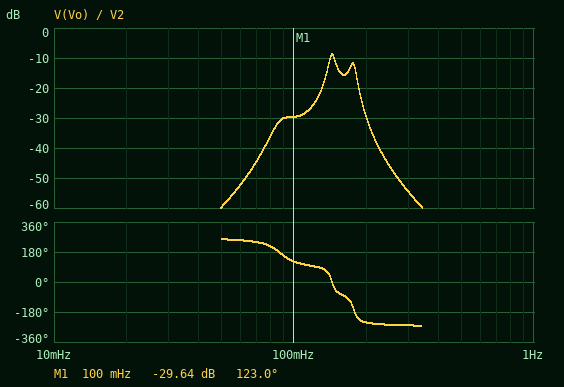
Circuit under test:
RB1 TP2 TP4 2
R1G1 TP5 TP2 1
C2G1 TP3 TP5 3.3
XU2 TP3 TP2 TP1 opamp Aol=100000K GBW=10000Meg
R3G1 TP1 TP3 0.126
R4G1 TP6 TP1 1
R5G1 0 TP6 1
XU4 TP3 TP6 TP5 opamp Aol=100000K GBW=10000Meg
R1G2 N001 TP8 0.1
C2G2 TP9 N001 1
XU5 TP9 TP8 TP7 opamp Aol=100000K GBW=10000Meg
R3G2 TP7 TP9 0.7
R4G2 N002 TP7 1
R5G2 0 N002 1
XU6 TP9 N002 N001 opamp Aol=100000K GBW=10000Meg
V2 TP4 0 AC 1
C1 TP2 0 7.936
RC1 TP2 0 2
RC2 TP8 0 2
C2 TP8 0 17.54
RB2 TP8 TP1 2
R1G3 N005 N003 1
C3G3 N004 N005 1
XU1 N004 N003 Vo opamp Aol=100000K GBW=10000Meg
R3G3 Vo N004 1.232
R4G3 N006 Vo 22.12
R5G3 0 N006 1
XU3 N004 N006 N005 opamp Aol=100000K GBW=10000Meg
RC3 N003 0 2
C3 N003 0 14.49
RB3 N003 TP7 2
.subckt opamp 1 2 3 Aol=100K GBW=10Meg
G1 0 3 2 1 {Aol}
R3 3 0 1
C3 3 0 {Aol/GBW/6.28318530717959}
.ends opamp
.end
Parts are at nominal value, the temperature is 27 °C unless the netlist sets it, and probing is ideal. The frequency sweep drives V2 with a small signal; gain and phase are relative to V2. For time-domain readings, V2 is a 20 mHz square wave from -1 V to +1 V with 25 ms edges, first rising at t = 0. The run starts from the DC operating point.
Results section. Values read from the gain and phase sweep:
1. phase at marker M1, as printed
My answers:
123.0 deg
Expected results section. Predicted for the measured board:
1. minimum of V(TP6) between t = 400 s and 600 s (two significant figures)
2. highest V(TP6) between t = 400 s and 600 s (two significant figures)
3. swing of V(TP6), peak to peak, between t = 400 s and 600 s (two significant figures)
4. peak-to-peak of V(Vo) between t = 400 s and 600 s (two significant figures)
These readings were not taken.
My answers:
-170 mV
170 mV
340 mV
140 mV
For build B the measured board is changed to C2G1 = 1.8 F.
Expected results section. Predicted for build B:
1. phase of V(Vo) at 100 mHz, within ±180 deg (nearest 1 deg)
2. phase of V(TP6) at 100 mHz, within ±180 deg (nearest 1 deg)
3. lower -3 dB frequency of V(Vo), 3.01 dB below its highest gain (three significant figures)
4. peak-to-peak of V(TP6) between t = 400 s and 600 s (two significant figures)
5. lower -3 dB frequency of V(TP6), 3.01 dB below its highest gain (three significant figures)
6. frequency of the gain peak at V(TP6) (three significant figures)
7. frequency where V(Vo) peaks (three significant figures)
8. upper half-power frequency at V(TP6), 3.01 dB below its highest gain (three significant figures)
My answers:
-124 deg
64 deg
139 mHz
250 mV
109 mHz
119 mHz
144 mHz
129 mHz
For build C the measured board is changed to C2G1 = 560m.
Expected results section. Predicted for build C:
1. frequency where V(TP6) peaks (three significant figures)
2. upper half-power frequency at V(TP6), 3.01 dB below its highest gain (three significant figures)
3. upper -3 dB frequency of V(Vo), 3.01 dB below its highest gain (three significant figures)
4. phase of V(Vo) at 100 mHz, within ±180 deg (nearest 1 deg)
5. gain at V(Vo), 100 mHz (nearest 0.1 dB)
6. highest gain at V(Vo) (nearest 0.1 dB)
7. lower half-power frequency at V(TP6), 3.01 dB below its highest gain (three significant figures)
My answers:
213 mHz
223 mHz
183 mHz
-101 deg
-50.9 dB
-7.4 dB
203 mHz
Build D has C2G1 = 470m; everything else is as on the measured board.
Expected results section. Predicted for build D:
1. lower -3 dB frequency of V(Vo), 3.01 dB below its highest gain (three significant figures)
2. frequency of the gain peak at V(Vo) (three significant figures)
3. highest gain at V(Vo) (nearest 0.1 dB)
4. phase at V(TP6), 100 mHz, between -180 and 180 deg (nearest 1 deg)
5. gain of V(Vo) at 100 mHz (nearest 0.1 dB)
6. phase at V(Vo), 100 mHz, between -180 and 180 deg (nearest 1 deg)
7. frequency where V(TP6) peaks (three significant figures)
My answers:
171 mHz
177 mHz
-11.5 dB
87 deg
-52.8 dB
-100 deg
232 mHz
